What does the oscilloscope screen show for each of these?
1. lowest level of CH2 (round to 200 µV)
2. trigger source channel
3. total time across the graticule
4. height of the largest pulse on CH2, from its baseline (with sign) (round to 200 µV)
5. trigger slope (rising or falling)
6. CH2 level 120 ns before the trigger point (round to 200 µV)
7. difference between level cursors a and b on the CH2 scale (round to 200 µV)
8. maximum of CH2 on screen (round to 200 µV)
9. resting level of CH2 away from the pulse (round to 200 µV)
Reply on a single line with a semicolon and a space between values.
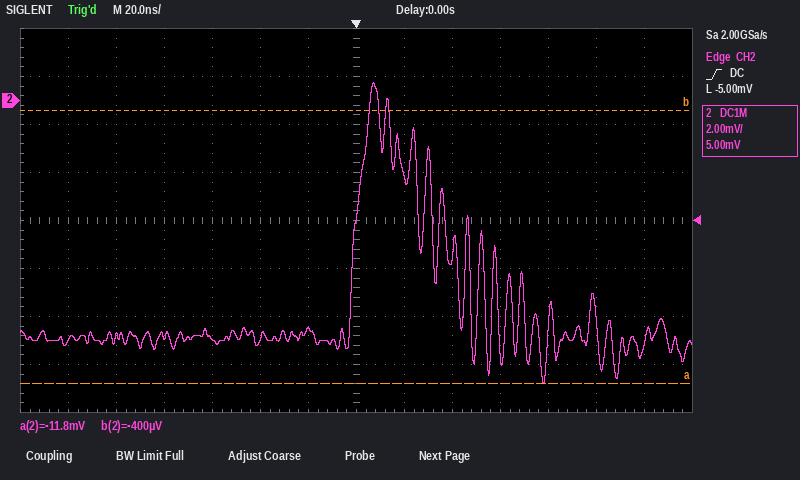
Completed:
-11.8 mV; CH2; 280 ns; +10.6 mV; rising; -10.0 mV; 11.4 mV; 800 µV; -9.8 mV
